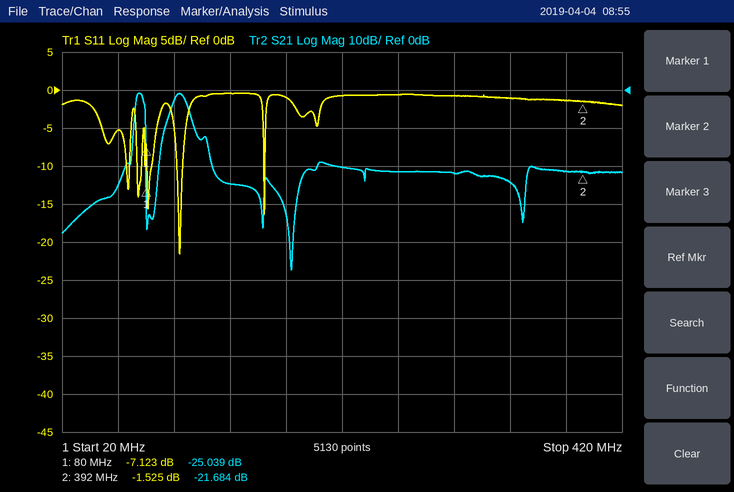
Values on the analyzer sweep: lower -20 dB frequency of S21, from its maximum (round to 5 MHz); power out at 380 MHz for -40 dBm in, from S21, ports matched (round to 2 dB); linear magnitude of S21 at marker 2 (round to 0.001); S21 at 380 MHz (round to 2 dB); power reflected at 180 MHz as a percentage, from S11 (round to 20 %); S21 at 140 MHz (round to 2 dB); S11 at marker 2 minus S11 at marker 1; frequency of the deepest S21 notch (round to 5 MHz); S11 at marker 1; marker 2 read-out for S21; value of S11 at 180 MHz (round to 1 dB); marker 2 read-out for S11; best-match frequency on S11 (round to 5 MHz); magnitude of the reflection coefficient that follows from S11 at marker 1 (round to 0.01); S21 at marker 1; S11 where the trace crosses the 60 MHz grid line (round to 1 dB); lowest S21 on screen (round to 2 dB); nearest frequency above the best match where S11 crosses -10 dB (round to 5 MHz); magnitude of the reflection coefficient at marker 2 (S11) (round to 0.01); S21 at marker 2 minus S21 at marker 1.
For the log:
65 MHz
-62 dBm
0.082
-22 dB
80 %
-24 dB
5.598 dB
185 MHz
-7.123 dB
-21.684 dB
-1 dB
-1.525 dB
105 MHz
0.44
-25.039 dB
-5 dB
-48 dB
105 MHz
0.84
3.355 dB
